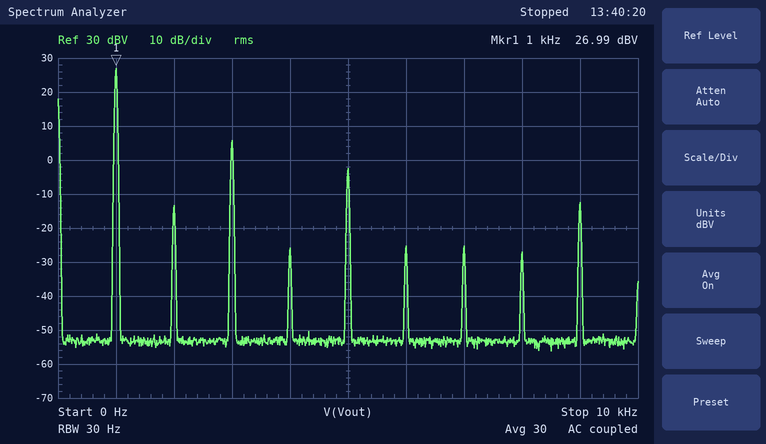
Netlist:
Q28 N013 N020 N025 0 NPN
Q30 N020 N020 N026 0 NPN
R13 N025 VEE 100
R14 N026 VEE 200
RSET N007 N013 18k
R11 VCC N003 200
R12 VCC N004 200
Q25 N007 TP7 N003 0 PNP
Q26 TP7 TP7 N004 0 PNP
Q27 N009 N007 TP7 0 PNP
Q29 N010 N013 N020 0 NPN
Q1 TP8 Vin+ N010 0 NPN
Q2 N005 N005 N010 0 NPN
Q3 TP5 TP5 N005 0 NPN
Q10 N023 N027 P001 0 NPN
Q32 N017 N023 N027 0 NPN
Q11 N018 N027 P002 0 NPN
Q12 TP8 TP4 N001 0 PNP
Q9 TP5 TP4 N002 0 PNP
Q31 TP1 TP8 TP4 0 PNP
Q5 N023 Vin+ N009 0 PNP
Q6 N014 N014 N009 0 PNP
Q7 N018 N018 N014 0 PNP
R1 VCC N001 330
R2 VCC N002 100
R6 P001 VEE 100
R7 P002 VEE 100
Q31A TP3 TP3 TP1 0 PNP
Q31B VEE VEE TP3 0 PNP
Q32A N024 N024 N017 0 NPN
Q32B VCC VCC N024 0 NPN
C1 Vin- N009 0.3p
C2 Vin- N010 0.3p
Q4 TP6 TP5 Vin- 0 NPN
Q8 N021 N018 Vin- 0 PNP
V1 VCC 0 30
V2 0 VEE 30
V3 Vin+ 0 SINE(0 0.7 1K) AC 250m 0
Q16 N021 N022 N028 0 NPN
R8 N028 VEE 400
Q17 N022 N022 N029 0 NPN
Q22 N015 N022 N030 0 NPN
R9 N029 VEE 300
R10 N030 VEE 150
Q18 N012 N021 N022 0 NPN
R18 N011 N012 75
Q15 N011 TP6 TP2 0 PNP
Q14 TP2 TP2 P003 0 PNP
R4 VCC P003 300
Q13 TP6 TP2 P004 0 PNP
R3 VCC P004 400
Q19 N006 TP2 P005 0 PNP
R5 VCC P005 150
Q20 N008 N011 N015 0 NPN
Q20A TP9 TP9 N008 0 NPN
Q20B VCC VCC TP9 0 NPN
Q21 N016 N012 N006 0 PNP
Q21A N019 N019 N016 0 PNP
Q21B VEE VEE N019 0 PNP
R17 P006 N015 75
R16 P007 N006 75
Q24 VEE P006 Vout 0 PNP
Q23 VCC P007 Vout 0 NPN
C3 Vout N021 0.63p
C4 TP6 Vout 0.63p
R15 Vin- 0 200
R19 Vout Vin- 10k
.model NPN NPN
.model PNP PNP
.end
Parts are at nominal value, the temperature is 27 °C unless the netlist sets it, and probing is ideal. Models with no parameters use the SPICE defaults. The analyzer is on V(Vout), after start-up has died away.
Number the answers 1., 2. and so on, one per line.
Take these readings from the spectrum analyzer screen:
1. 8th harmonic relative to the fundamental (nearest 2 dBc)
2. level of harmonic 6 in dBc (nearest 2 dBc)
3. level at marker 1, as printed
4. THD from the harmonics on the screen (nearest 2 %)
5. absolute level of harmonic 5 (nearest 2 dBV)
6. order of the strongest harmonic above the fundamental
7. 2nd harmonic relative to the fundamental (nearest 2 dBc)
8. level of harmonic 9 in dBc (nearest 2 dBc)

1. -54 dBc
2. -52 dBc
3. 26.99 dBV
4. 10 %
5. -2 dBV
6. 3
7. -40 dBc
8. -40 dBc
